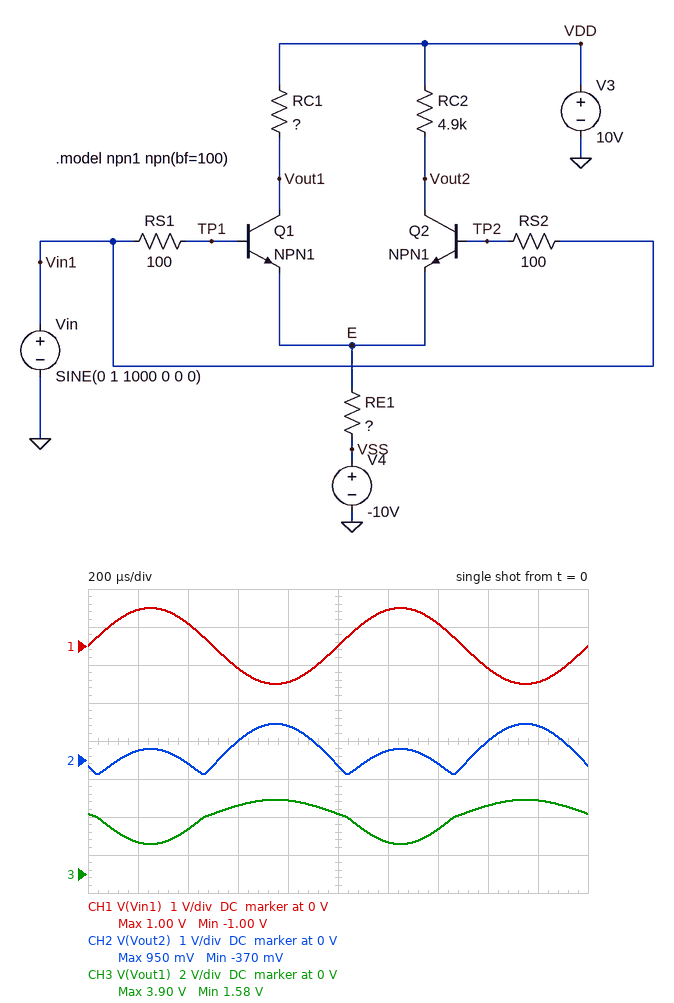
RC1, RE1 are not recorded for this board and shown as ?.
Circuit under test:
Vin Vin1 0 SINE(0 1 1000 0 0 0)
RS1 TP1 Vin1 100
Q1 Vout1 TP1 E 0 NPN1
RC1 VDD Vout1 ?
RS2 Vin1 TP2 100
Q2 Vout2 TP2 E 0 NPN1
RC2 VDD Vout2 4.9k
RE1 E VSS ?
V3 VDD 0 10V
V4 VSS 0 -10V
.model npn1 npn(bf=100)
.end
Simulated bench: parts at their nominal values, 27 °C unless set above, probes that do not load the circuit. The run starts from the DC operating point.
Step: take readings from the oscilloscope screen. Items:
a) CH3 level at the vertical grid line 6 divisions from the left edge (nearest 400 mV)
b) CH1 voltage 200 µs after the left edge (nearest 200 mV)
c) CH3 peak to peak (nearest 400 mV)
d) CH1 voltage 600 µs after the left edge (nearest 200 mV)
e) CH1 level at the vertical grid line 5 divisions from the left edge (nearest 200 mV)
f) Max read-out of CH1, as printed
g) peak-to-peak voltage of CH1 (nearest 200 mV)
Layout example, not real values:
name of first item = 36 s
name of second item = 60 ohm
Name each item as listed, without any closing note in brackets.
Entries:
CH3 level at the vertical grid line 6 divisions from the left edge = 1.6 V
CH1 voltage 200 µs after the left edge = 1.0 V
CH3 peak to peak = 2.4 V
CH1 voltage 600 µs after the left edge = -600 mV
CH1 level at the vertical grid line 5 divisions from the left edge = 0 V
Max read-out of CH1, as printed = 1.00 V
peak-to-peak voltage of CH1 = 2.0 V
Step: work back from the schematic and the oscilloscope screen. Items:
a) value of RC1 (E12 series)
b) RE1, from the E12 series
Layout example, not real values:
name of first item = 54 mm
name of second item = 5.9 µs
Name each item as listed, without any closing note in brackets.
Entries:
value of RC1 = 3.3 kΩ
RE1, from the E12 series = 2.2 kΩ
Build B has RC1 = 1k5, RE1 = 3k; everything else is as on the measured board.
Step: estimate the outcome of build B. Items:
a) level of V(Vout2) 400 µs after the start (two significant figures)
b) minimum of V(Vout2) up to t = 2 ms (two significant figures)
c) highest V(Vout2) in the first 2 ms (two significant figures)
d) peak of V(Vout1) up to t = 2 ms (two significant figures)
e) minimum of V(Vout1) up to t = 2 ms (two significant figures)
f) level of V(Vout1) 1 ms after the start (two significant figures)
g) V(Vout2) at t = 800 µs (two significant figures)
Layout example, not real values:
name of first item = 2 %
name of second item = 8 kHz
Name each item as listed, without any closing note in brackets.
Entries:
level of V(Vout2) 400 µs after the start = 2.1 V
minimum of V(Vout2) up to t = 2 ms = 1.7 V
highest V(Vout2) in the first 2 ms = 3.4 V
peak of V(Vout1) up to t = 2 ms = 8.0 V
minimum of V(Vout1) up to t = 2 ms = 7.5 V
level of V(Vout1) 1 ms after the start = 7.7 V
V(Vout2) at t = 800 µs = 3.3 V
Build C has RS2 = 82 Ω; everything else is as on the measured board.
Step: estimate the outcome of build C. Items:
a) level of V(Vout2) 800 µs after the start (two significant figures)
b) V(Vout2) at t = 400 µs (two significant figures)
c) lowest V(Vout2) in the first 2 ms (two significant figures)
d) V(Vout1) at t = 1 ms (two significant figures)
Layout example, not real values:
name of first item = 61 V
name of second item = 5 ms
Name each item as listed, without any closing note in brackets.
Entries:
level of V(Vout2) 800 µs after the start = 840 mV
V(Vout2) at t = 400 µs = -100 mV
lowest V(Vout2) in the first 2 ms = -410 mV
V(Vout1) at t = 1 ms = 3.2 V
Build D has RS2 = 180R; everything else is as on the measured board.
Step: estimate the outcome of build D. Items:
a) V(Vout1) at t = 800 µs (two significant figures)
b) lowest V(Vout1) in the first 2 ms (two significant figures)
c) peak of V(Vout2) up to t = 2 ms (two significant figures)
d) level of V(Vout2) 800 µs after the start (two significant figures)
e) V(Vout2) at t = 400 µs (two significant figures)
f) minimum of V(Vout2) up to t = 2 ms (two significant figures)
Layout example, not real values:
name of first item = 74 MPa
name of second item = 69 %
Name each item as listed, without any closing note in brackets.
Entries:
V(Vout1) at t = 800 µs = 3.7 V
lowest V(Vout1) in the first 2 ms = 1.5 V
peak of V(Vout2) up to t = 2 ms = 1.2 V
level of V(Vout2) 800 µs after the start = 1.1 V
V(Vout2) at t = 400 µs = -72 mV
minimum of V(Vout2) up to t = 2 ms = -220 mV
